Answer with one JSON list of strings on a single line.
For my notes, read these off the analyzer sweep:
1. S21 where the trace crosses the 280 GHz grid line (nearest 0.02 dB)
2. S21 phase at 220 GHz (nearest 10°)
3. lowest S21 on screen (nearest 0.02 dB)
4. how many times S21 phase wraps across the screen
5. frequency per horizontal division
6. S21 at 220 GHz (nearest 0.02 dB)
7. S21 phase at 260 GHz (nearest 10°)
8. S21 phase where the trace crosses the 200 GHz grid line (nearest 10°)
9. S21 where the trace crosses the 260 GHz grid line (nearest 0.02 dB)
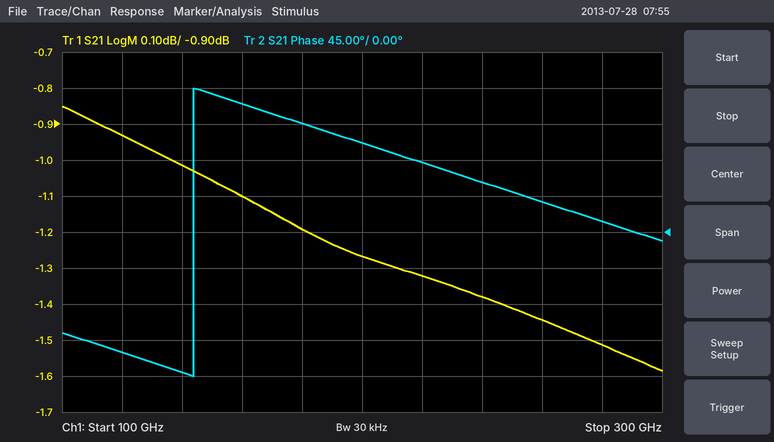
["-1.52 dB", "90°", "-1.58 dB", "1", "20 GHz", "-1.32 dB", "40°", "110°", "-1.44 dB"]
